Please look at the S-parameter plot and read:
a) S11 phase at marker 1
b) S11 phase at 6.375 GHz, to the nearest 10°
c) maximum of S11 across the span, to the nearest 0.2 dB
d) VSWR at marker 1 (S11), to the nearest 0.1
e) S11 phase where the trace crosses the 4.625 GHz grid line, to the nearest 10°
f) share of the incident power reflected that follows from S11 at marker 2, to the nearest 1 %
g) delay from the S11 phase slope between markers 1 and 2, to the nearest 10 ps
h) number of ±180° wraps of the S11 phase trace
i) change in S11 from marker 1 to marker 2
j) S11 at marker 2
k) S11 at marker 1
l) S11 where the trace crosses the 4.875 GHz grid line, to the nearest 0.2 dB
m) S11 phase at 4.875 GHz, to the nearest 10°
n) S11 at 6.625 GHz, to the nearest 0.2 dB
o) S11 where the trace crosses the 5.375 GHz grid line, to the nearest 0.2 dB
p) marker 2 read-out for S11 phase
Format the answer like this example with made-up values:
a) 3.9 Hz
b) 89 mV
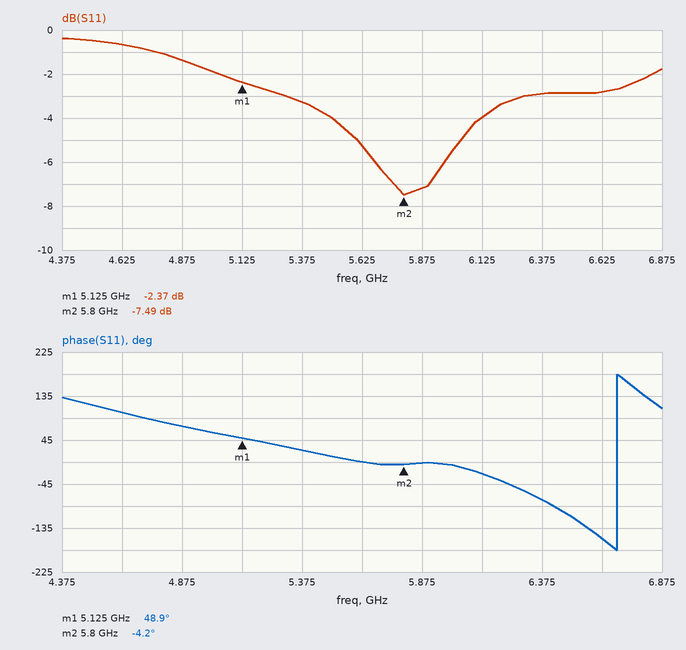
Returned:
a) 48.9°
b) -80°
c) -0.4 dB
d) 7.4
e) 100°
f) 18 %
g) 220 ps
h) 1
i) -5.12 dB
j) -7.49 dB
k) -2.37 dB
l) -1.4 dB
m) 70°
n) -2.8 dB
o) -3.2 dB
p) -4.2°
